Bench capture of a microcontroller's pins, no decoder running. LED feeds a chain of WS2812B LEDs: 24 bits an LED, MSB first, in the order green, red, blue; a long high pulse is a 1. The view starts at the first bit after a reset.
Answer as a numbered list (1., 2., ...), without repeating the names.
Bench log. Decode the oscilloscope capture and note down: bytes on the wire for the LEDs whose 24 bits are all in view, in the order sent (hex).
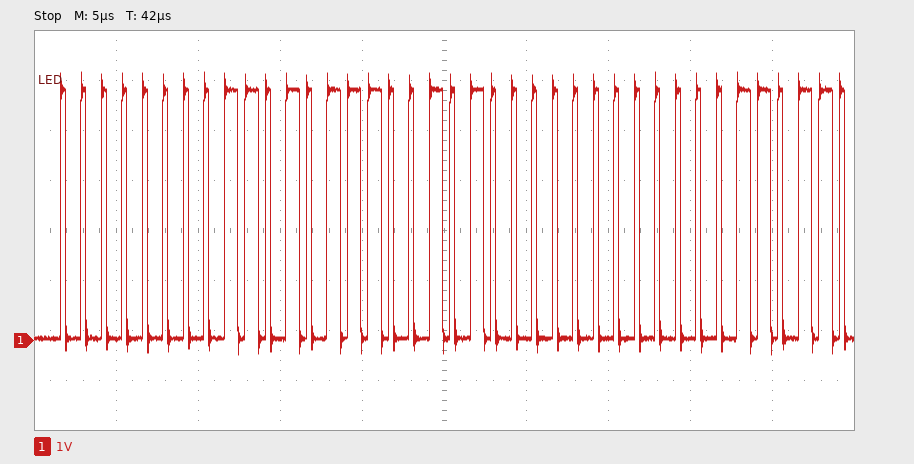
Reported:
1. 00 D7 28
